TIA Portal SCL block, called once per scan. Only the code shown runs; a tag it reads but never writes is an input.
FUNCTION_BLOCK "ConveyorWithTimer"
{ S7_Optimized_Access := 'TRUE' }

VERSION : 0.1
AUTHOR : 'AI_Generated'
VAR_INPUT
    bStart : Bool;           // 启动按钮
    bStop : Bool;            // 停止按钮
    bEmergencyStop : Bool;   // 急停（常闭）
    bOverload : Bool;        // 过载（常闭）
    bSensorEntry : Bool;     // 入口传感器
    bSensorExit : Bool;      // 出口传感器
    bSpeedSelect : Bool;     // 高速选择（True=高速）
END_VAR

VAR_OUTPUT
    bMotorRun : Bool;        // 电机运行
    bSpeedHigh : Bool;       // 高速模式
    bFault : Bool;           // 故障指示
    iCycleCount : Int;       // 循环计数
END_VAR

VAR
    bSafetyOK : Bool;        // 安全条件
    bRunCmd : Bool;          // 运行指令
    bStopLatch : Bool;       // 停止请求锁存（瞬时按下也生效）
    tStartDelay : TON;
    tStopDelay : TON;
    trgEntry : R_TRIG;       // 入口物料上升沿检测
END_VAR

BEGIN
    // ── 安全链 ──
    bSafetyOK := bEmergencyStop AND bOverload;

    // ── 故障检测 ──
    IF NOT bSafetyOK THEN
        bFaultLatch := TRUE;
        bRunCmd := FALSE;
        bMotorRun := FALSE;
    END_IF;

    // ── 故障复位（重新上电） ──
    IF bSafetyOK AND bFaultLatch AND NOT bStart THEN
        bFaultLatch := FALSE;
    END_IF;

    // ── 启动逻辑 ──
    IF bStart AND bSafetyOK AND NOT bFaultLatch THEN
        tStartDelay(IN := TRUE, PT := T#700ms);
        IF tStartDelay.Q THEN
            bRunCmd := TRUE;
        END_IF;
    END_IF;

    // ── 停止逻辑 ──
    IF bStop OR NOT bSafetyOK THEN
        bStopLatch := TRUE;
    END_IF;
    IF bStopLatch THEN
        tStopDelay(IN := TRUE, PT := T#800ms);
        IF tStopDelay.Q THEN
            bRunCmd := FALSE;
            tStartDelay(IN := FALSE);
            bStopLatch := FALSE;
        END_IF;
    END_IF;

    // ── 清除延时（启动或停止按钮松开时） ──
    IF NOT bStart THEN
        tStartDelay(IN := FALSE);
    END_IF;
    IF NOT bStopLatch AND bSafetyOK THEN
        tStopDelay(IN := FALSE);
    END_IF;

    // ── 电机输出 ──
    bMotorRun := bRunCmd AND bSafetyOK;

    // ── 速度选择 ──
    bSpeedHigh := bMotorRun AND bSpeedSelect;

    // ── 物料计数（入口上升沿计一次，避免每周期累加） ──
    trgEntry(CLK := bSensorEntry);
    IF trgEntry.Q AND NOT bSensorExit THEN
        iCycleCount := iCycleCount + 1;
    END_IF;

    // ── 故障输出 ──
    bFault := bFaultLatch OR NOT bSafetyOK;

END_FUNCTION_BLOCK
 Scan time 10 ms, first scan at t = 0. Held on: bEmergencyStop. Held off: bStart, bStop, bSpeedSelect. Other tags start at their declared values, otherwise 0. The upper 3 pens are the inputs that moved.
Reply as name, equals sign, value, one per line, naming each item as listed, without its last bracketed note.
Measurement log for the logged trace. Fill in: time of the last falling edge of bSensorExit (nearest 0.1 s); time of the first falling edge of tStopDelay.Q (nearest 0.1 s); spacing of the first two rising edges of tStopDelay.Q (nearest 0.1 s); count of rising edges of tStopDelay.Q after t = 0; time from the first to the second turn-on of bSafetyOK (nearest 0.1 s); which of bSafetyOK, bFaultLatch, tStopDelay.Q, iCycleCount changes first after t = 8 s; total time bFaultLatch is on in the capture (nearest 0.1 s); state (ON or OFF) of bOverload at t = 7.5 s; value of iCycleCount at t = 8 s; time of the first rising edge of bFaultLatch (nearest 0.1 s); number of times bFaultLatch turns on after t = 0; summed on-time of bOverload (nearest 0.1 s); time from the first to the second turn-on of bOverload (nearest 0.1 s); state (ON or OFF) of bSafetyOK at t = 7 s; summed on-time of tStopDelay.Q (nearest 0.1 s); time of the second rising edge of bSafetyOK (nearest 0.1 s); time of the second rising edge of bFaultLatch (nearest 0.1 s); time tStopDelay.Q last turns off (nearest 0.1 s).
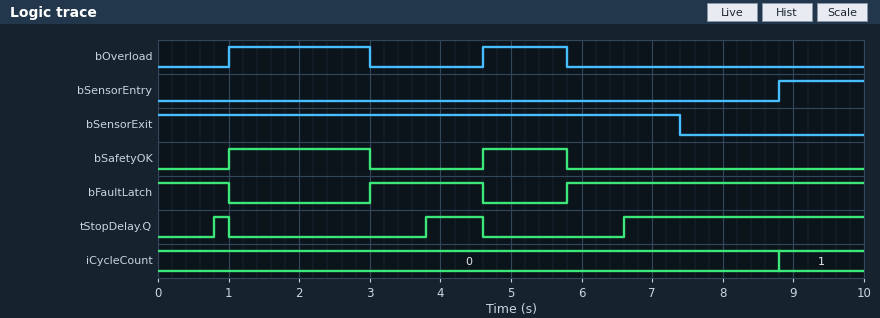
time of the last falling edge of bSensorExit = 7.4 s
time of the first falling edge of tStopDelay.Q = 1.0 s
spacing of the first two rising edges of tStopDelay.Q = 3.0 s
count of rising edges of tStopDelay.Q after t = 0 = 3
time from the first to the second turn-on of bSafetyOK = 3.6 s
which of bSafetyOK, bFaultLatch, tStopDelay.Q, iCycleCount changes first after t = 8 s = iCycleCount
total time bFaultLatch is on in the capture = 6.8 s
state (ON or OFF) of bOverload at t = 7.5 s = OFF
value of iCycleCount at t = 8 s = 0
time of the first rising edge of bFaultLatch = 3.0 s
number of times bFaultLatch turns on after t = 0 = 2
summed on-time of bOverload = 3.2 s
time from the first to the second turn-on of bOverload = 3.6 s
state (ON or OFF) of bSafetyOK at t = 7 s = OFF
summed on-time of tStopDelay.Q = 4.4 s
time of the second rising edge of bSafetyOK = 4.6 s
time of the second rising edge of bFaultLatch = 5.8 s
time tStopDelay.Q last turns off = 4.6 s
